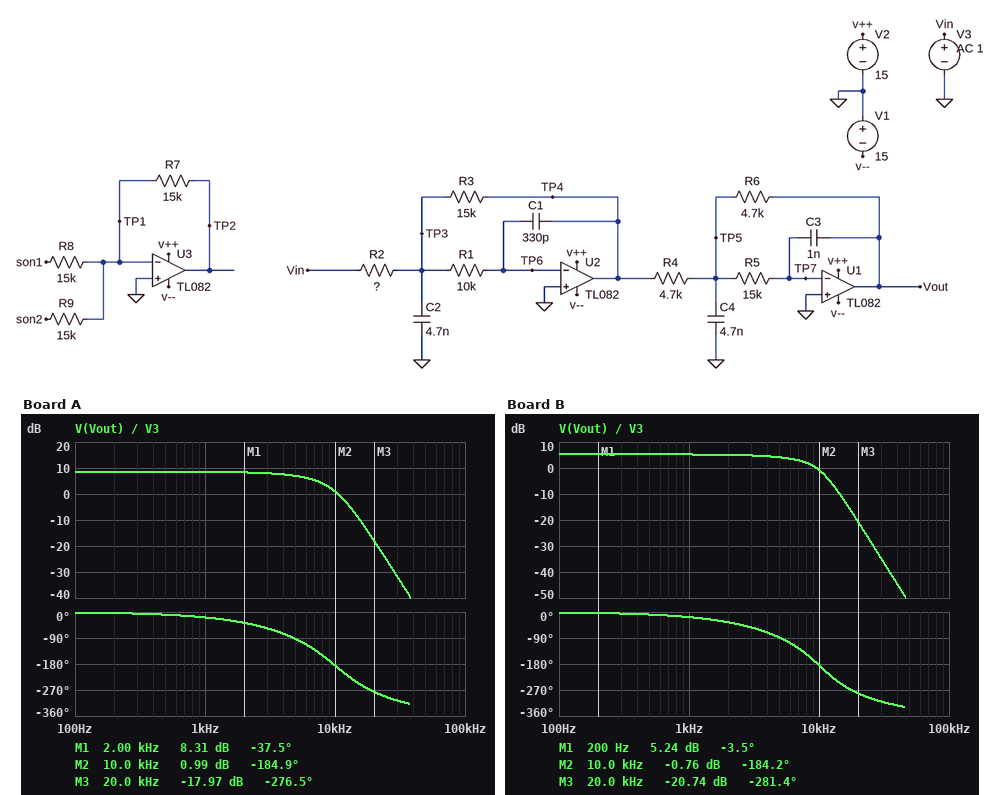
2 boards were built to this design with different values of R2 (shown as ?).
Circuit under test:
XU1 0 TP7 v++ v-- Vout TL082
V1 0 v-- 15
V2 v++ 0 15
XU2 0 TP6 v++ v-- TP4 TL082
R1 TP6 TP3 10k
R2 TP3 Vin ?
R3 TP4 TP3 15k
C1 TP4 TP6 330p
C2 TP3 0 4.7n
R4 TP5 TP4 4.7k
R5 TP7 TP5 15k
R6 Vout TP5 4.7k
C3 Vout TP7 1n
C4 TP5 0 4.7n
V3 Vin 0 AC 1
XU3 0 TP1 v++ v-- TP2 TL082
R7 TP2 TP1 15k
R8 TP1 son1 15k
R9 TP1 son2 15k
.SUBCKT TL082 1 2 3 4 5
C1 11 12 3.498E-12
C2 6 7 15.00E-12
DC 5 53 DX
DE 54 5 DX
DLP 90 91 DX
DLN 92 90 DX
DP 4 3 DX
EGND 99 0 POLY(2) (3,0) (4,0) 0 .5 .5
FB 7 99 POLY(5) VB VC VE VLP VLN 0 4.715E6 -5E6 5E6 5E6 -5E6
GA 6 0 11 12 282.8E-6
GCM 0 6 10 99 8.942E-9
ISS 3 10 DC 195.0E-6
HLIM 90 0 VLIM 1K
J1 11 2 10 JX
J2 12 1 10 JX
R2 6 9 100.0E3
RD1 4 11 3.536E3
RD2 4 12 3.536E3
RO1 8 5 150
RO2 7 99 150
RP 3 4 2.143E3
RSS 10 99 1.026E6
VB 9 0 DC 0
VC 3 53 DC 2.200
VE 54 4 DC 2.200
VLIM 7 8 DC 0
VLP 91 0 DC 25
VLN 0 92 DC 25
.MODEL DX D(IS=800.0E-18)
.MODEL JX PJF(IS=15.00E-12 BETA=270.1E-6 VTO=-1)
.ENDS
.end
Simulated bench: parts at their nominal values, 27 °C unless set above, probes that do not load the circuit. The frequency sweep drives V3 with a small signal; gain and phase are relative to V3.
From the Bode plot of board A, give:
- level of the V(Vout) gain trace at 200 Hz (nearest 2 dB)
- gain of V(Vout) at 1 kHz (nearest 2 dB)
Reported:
8 dB
8 dB
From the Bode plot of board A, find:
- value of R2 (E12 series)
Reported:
5.6 kΩ
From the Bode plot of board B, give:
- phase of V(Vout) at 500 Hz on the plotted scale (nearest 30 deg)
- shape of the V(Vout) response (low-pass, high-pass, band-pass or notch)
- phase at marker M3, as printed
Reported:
0 deg
low-pass
-281.4 deg
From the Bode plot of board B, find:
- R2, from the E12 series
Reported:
8.2 kΩ
